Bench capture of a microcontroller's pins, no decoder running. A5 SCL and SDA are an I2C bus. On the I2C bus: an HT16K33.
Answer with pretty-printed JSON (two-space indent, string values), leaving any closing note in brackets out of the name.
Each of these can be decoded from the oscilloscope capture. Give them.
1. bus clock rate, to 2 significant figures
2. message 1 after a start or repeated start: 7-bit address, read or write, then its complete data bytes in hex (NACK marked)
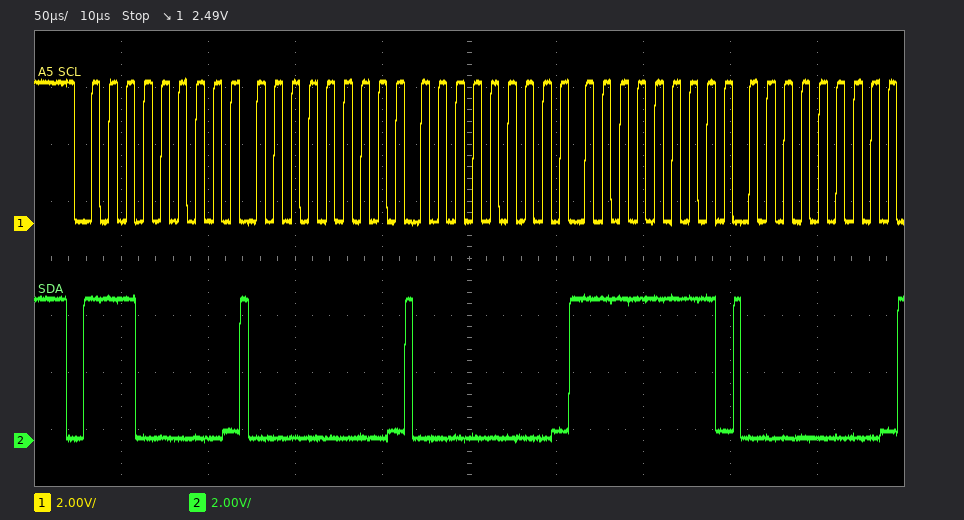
{
  "bus clock rate, to 2 significant figures": "100 kHz",
  "message 1 after a start or repeated start: 7-bit address, read or write, then its complete data bytes in hex": "0x70 write: 00 00 FF 00"
}
